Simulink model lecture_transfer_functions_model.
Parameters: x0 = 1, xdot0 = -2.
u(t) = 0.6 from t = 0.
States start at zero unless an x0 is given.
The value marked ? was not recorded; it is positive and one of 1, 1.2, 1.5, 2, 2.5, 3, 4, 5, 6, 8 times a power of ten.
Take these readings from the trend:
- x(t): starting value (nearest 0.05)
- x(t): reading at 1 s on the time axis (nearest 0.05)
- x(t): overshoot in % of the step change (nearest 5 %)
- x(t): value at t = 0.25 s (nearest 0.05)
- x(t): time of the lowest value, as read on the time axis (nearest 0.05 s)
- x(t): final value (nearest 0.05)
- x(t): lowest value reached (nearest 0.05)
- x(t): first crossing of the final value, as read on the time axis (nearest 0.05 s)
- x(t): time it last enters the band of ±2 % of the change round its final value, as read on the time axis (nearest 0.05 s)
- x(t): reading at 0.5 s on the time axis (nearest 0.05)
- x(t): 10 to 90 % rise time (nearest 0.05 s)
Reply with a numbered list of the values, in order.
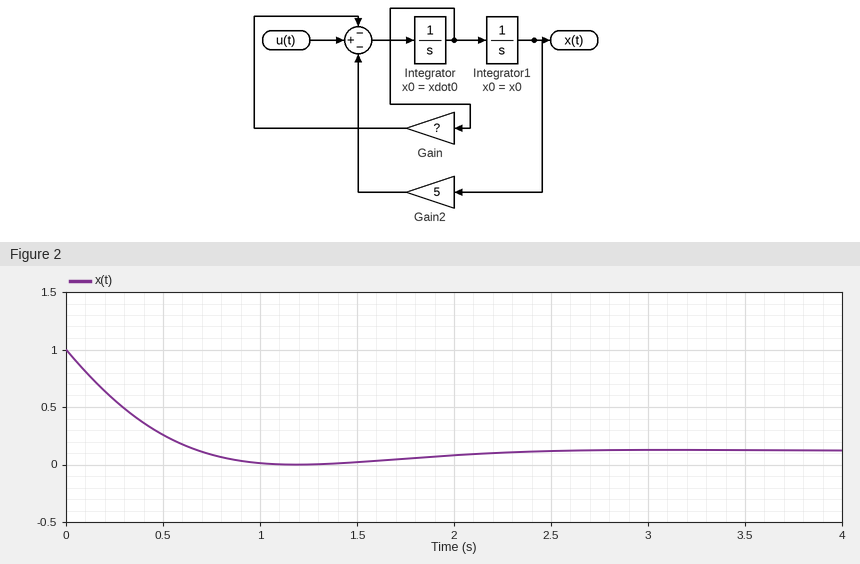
1. 1.00
2. 0.00
3. 15 %
4. 0.55
5. 1.20 s
6. 0.10
7. 0.00
8. 0.70 s
9. 2.25 s
10. 0.25
11. 0.50 s
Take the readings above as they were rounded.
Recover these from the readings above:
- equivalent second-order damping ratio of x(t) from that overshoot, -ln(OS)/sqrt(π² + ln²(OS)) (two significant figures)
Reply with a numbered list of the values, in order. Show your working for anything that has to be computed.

1. ln(0.15) = -1.897; 1.897 / sqrt(9.870 + 3.599) = 0.52
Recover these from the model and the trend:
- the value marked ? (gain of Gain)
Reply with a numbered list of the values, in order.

1. 3
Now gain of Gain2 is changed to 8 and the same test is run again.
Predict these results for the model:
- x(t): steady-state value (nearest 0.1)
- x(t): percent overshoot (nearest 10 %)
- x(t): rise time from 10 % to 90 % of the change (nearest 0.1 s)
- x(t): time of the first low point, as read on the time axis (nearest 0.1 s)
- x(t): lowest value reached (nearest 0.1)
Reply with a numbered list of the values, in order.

1. 0.1
2. 20 %
3. 0.4 s
4. 1.0 s
5. -0.1
